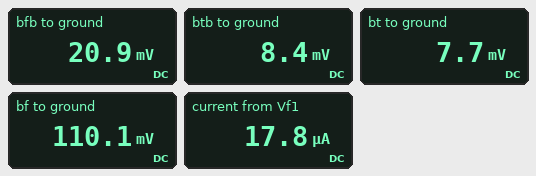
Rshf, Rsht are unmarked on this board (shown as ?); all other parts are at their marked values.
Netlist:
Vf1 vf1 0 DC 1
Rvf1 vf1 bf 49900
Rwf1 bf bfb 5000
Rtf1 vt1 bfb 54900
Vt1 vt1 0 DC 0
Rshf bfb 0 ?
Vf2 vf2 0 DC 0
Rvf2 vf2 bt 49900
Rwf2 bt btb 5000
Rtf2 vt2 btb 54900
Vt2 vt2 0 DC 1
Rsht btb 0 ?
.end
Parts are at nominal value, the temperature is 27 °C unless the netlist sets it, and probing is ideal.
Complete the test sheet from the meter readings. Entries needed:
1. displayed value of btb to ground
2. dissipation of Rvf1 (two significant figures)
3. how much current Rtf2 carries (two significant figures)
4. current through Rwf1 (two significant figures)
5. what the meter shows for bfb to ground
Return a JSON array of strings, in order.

["8.4 mV", "16 µW", "18 µA", "18 µA", "20.9 mV"]
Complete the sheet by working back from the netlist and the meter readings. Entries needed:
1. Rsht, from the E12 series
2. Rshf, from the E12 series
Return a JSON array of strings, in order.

["470 Ω", "1.2 kΩ"]
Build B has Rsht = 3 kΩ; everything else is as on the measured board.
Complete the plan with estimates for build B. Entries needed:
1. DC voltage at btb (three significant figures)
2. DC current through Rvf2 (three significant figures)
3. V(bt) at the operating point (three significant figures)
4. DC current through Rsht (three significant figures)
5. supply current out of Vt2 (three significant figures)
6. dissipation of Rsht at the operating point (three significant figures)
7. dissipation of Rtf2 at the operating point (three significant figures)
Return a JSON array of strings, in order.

["49.3 mV", "897 nA", "44.8 mV", "16.4 µA", "17.3 µA", "809 nW", "16.5 µW"]
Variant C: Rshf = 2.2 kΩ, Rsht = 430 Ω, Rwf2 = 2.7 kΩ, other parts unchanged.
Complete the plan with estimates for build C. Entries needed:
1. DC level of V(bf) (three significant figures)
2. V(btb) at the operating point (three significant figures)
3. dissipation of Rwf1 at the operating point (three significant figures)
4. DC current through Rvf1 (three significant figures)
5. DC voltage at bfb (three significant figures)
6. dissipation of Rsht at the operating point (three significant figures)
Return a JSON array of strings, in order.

["125 mV", "7.71 mV", "1.54 µW", "17.5 µA", "37.1 mV", "138 nW"]
